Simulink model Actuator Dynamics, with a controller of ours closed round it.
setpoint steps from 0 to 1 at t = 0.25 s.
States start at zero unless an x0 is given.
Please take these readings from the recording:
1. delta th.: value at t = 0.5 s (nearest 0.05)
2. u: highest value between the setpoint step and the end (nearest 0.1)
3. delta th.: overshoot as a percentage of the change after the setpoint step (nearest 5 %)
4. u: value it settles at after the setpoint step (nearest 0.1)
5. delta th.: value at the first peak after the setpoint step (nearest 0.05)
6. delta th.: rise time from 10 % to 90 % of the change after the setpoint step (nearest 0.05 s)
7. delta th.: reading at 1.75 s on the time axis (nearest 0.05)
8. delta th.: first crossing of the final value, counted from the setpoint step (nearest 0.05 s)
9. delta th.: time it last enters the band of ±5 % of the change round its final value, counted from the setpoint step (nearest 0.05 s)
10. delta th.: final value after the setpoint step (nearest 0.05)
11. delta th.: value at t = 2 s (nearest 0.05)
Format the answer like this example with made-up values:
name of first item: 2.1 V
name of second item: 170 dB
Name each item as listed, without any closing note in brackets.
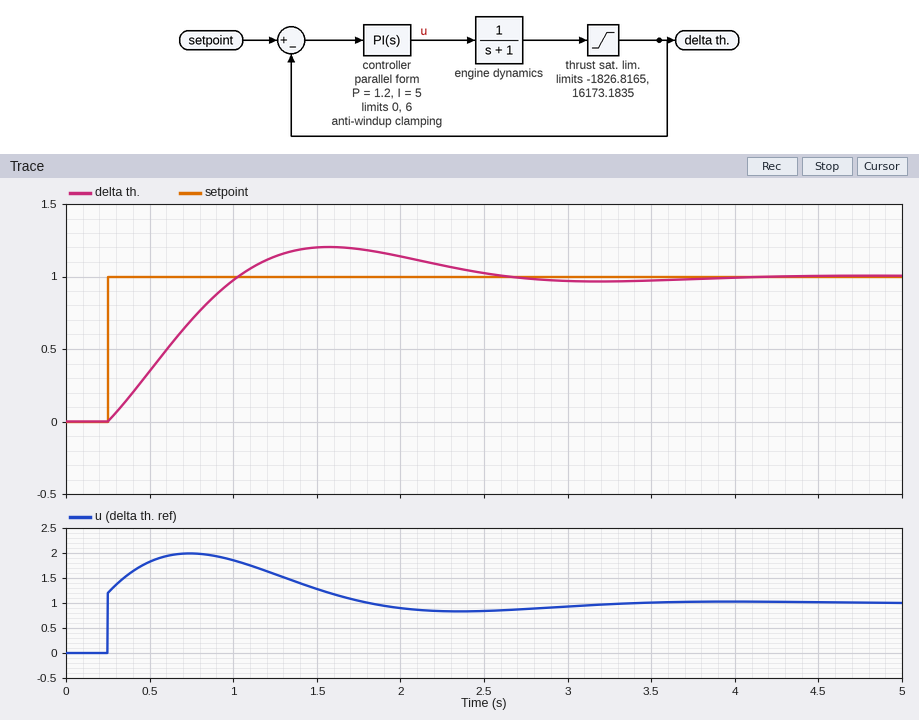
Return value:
delta th.: value at t = 0.5 s: 0.35
u: highest value between the setpoint step and the end: 2.0
delta th.: overshoot as a percentage of the change after the setpoint step: 20 %
u: value it settles at after the setpoint step: 1.0
delta th.: value at the first peak after the setpoint step: 1.20
delta th.: rise time from 10 % to 90 % of the change after the setpoint step: 0.60 s
delta th.: reading at 1.75 s on the time axis: 1.20
delta th.: first crossing of the final value, counted from the setpoint step: 0.80 s
delta th.: time it last enters the band of ±5 % of the change round its final value, counted from the setpoint step: 2.10 s
delta th.: final value after the setpoint step: 1.00
delta th.: value at t = 2 s: 1.15
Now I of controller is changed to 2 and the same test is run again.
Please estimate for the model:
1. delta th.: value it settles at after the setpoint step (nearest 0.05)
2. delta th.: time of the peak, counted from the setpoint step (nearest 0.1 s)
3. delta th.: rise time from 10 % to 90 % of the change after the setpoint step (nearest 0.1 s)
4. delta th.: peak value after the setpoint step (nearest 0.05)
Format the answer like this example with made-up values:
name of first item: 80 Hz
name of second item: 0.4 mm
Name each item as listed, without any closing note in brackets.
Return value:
delta th.: value it settles at after the setpoint step: 1.00
delta th.: time of the peak, counted from the setpoint step: 2.4 s
delta th.: rise time from 10 % to 90 % of the change after the setpoint step: 1.1 s
delta th.: peak value after the setpoint step: 1.05
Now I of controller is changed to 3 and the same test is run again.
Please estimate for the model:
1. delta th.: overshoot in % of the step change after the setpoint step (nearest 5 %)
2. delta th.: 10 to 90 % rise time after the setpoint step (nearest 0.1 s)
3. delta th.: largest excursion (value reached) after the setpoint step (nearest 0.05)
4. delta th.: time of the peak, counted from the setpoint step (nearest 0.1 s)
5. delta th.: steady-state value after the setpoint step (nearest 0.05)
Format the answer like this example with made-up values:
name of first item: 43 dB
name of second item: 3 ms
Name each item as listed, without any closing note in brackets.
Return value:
delta th.: overshoot in % of the step change after the setpoint step: 10 %
delta th.: 10 to 90 % rise time after the setpoint step: 0.8 s
delta th.: largest excursion (value reached) after the setpoint step: 1.10
delta th.: time of the peak, counted from the setpoint step: 1.8 s
delta th.: steady-state value after the setpoint step: 1.00
